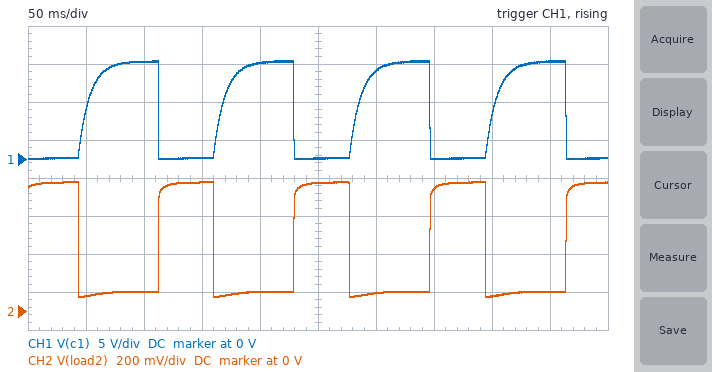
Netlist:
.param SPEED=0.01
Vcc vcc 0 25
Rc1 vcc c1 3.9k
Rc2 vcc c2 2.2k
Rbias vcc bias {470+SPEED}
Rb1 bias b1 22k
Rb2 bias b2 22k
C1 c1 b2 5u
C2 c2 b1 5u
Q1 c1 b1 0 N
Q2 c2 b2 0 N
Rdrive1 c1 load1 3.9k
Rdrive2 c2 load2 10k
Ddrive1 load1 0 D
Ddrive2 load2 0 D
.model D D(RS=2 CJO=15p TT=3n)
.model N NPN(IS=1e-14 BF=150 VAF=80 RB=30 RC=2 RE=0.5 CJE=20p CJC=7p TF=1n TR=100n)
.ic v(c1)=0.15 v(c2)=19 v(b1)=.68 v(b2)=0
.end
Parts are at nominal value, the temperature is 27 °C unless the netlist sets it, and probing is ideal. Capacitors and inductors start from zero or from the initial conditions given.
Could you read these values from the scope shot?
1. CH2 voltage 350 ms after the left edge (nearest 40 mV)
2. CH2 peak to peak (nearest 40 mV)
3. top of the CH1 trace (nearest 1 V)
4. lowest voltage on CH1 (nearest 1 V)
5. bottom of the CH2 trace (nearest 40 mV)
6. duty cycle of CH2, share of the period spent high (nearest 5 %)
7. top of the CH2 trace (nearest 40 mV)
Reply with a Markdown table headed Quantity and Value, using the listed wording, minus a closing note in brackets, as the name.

| Quantity | Value |
|---|---|
| CH2 voltage 350 ms after the left edge | 640 mV |
| CH2 peak to peak | 600 mV |
| top of the CH1 trace | 13 V |
| lowest voltage on CH1 | 0 V |
| bottom of the CH2 trace | 80 mV |
| duty cycle of CH2, share of the period spent high | 40 % |
| top of the CH2 trace | 680 mV |
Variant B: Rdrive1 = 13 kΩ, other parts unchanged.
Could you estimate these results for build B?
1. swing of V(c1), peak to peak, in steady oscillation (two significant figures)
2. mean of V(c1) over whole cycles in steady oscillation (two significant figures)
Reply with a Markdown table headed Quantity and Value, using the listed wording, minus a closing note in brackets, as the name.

| Quantity | Value |
|---|---|
| swing of V(c1), peak to peak, in steady oscillation | 19 V |
| mean of V(c1) over whole cycles in steady oscillation | 7.9 V |
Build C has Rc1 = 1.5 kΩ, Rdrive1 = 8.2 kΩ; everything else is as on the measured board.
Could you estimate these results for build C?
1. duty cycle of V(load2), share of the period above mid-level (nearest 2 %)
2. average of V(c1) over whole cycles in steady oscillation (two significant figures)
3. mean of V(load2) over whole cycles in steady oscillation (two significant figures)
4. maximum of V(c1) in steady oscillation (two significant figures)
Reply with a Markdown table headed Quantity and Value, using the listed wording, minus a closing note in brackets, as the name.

| Quantity | Value |
|---|---|
| duty cycle of V(load2), share of the period above mid-level | 50 % |
| average of V(c1) over whole cycles in steady oscillation | 9.6 V |
| mean of V(load2) over whole cycles in steady oscillation | 390 mV |
| maximum of V(c1) in steady oscillation | 21 V |
